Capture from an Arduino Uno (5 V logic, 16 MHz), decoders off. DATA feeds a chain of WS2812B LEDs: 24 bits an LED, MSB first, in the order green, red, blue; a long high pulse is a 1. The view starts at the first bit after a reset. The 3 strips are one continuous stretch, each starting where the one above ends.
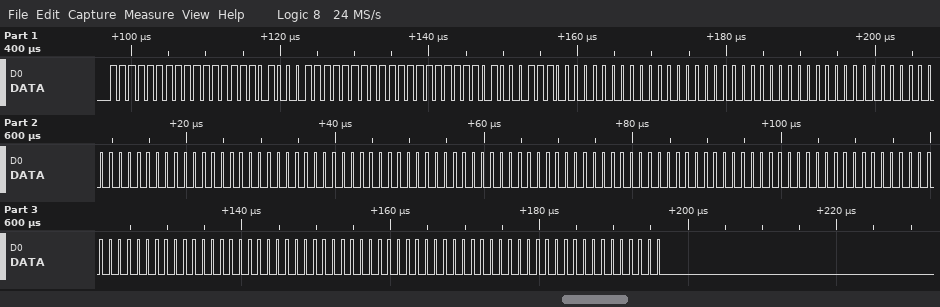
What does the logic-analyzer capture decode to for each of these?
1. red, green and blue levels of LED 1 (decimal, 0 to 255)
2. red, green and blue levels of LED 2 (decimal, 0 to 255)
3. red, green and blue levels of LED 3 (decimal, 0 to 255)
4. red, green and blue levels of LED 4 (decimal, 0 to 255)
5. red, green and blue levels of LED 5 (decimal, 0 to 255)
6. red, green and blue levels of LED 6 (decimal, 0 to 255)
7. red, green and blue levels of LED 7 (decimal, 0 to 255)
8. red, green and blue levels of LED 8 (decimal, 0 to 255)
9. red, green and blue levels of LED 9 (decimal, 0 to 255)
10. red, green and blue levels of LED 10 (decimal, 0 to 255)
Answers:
255, 255, 71
255, 255, 71
0, 0, 0
0, 0, 0
0, 0, 0
0, 0, 0
0, 0, 0
0, 0, 0
0, 0, 0
0, 0, 0
